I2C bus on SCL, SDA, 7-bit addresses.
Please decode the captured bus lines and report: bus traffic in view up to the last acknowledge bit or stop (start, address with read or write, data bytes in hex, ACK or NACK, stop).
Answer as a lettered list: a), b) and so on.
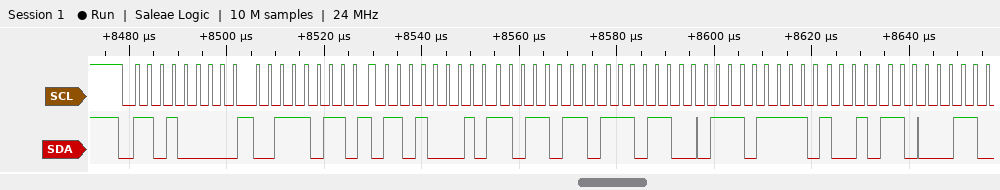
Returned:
a) start, address 68 write ACK, 3B ACK, repeated start, address 68 read ACK, DB ACK, EC ACK, EF ACK, 96 ACK
